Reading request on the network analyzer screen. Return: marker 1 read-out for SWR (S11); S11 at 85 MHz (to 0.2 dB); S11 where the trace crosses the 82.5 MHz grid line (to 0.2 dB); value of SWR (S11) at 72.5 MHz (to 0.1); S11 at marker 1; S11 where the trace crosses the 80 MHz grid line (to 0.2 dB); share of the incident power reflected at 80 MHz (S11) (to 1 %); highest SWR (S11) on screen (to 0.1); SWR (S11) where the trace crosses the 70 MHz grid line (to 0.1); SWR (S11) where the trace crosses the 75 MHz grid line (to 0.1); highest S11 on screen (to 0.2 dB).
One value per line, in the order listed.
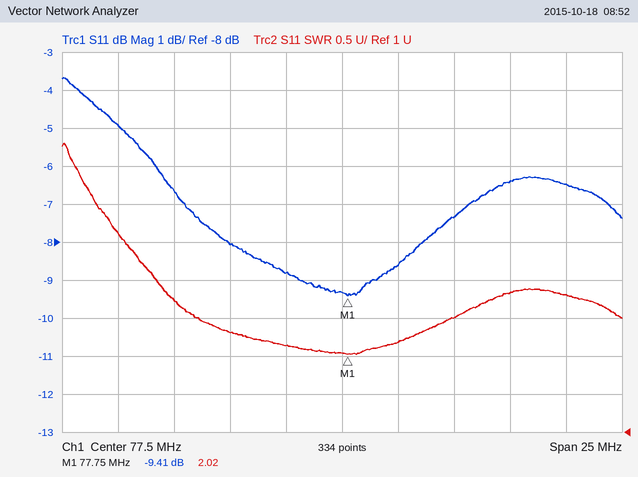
2.02
-6.4 dB
-7.4 dB
2.3
-9.41 dB
-8.6 dB
14 %
4.8
2.7
2.1
-3.6 dB
